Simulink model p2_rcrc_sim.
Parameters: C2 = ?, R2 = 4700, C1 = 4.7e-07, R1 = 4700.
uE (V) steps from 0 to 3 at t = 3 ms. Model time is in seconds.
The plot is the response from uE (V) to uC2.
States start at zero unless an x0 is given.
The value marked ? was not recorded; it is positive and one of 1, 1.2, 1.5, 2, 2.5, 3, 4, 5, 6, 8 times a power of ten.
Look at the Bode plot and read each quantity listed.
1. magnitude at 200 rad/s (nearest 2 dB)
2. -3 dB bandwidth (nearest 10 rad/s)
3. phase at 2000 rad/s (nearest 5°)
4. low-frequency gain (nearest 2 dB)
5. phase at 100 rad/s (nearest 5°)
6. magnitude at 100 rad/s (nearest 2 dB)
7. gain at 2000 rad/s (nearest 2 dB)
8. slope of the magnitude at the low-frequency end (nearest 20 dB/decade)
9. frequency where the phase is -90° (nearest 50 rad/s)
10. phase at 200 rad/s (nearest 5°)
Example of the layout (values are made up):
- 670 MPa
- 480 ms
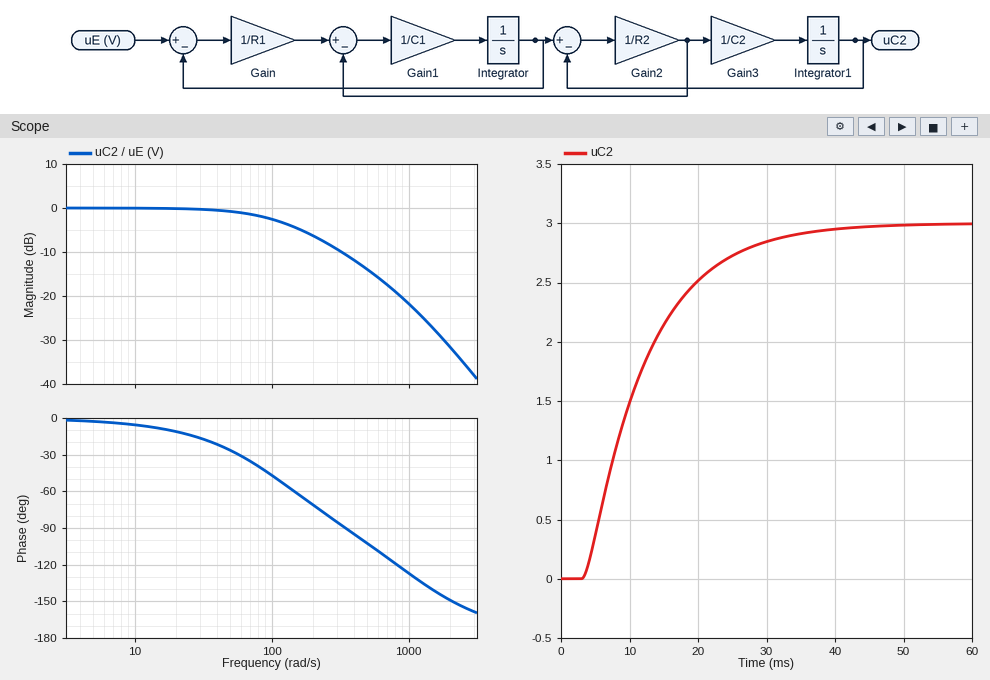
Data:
- -6 dB
- 110 rad/s
- -150°
- 0 dB
- -45°
- -2 dB
- -32 dB
- 0 dB/decade
- 350 rad/s
- -70°
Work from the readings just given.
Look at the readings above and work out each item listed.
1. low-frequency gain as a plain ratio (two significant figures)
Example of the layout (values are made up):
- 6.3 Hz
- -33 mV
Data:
- 1.0
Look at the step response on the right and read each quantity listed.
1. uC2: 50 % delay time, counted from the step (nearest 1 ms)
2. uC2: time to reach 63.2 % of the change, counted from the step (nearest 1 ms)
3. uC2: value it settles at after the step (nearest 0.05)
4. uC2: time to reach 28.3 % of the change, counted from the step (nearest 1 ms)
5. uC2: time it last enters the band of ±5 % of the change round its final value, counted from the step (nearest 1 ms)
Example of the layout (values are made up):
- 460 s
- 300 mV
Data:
- 7 ms
- 10 ms
- 3.00
- 4 ms
- 27 ms
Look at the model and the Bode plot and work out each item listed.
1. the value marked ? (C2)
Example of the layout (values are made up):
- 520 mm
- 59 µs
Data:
- 8e-07
